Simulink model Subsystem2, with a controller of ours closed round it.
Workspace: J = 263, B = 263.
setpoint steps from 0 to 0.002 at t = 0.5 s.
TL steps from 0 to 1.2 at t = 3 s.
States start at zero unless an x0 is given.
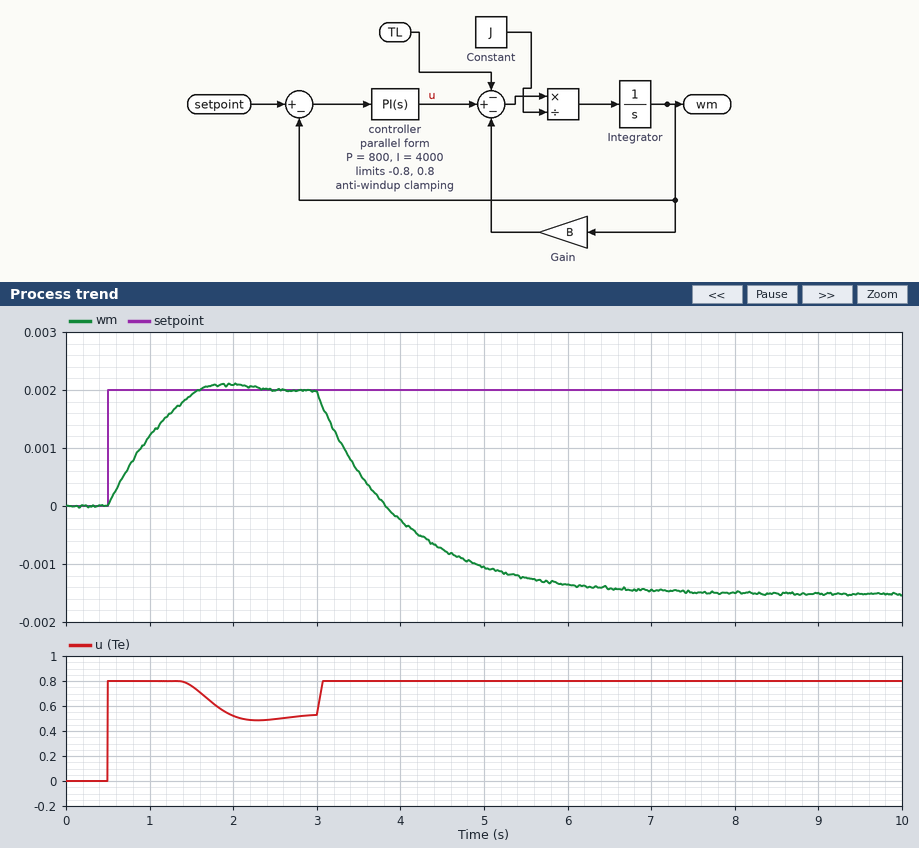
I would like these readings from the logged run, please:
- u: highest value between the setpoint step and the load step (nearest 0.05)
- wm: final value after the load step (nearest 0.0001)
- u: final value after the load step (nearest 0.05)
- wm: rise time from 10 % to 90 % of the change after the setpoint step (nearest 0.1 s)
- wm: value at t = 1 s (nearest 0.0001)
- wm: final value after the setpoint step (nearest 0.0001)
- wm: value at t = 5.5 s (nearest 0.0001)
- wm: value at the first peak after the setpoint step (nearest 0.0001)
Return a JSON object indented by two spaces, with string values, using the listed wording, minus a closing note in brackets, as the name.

{
  "u: highest value between the setpoint step and the load step": "0.80",
  "wm: final value after the load step": "-0.0015",
  "u: final value after the load step": "0.80",
  "wm: rise time from 10 % to 90 % of the change after the setpoint step": "0.8 s",
  "wm: value at t = 1 s": "0.0012",
  "wm: final value after the setpoint step": "0.0020",
  "wm: value at t = 5.5 s": "-0.0012",
  "wm: value at the first peak after the setpoint step": "0.0021"
}
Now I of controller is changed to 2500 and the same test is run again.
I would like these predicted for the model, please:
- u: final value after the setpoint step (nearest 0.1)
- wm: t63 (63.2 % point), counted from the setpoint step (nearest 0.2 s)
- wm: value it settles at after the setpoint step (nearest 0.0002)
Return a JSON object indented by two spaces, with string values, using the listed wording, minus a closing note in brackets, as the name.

{
  "u: final value after the setpoint step": "0.5",
  "wm: t63 (63.2 % point), counted from the setpoint step": "0.6 s",
  "wm: value it settles at after the setpoint step": "0.0020"
}
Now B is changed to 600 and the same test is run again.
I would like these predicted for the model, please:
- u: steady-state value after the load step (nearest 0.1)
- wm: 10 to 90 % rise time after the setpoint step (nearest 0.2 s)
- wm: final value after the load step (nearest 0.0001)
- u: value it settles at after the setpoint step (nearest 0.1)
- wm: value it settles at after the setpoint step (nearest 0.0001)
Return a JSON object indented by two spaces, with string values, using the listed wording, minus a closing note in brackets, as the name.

{
  "u: steady-state value after the load step": "0.8",
  "wm: 10 to 90 % rise time after the setpoint step": "1.0 s",
  "wm: final value after the load step": "-0.0007",
  "u: value it settles at after the setpoint step": "0.8",
  "wm: value it settles at after the setpoint step": "0.0013"
}
